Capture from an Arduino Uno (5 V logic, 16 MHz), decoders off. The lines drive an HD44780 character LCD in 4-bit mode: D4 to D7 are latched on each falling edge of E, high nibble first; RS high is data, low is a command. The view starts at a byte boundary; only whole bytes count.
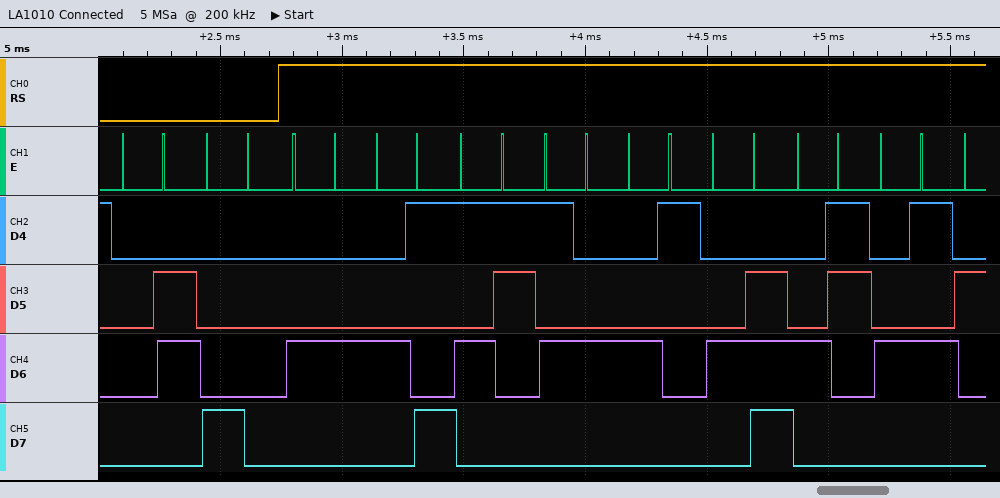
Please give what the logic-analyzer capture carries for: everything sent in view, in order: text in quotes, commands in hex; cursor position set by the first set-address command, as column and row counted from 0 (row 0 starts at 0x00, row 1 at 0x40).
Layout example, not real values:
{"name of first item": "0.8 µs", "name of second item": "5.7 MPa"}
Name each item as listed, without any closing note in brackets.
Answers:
{"everything sent in view, in order: text in quotes, commands in hex": "0x06 0x80 \"DISTANCE\"", "cursor position set by the first set-address command, as column and row counted from 0": "column 0, row 0"}
